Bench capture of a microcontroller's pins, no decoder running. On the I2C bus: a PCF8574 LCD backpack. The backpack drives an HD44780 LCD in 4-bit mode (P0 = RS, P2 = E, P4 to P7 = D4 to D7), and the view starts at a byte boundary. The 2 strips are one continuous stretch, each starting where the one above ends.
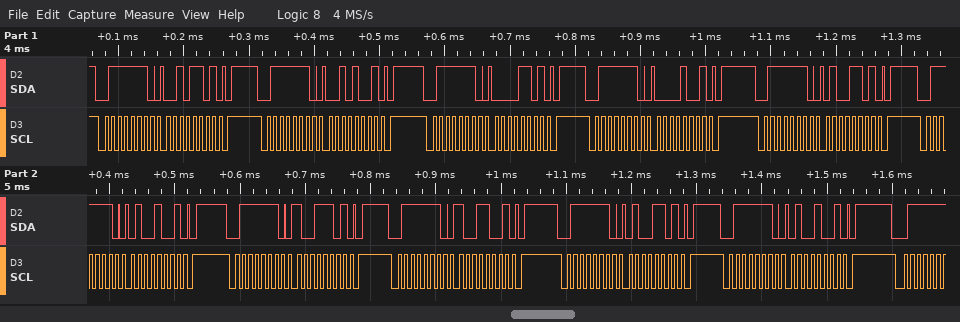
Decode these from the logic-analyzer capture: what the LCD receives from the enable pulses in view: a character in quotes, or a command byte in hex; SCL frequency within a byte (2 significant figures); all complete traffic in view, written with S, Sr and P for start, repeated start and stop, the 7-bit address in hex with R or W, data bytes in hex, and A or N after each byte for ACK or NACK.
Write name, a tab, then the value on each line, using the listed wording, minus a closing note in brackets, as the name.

what the LCD receives from the enable pulses in view: a character in quotes, or a command byte in hex	' ' 'I'
SCL frequency within a byte	100 kHz
all complete traffic in view, written with S, Sr and P for start, repeated start and stop, the 7-bit address in hex with R or W, data bytes in hex, and A or N after each byte for ACK or NACK	S 3FW A 2D A P S 3FW A 29 A P S 3FW A 0D A P S 3FW A 09 A P S 3FW A 4D A P S 3FW A 49 A P S 3FW A 9D A P S 3FW A 99 A P S 3FW A 4D A P S 3FW A 49 A P
